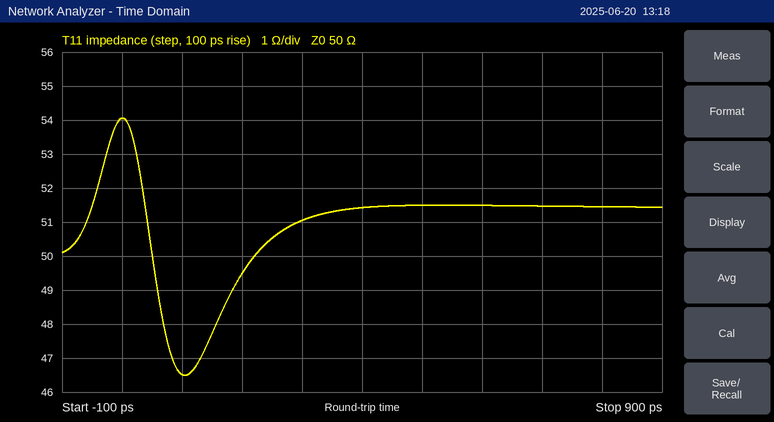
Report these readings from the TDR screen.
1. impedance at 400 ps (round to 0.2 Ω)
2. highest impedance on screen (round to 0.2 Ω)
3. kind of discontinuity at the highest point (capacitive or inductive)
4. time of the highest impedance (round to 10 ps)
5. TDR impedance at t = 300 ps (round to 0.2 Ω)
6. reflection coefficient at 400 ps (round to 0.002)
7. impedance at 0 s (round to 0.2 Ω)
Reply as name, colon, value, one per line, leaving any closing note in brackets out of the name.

impedance at 400 ps: 51.4 Ω
highest impedance on screen: 54.0 Ω
kind of discontinuity at the highest point: inductive
time of the highest impedance: 0 ps
TDR impedance at t = 300 ps: 51.0 Ω
reflection coefficient at 400 ps: +0.014
impedance at 0 s: 54.0 Ω
